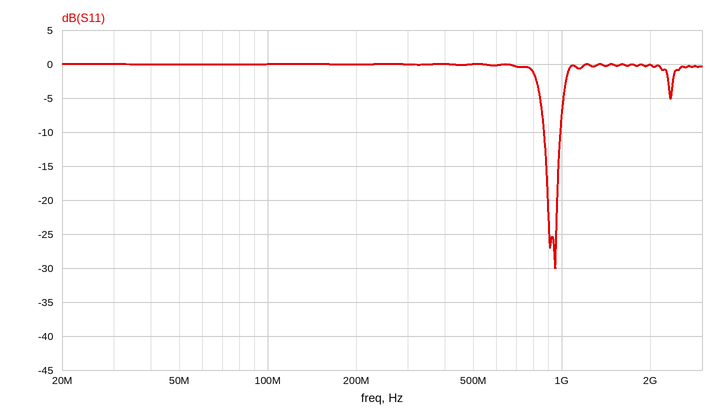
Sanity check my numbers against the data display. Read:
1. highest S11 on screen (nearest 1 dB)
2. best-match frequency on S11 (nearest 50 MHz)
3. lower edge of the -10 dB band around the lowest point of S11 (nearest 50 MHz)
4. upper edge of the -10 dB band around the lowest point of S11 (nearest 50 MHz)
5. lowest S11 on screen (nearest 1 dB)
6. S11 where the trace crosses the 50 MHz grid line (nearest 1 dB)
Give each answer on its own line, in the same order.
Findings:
0 dB
950 MHz
850 MHz
1.00 GHz
-30 dB
0 dB
